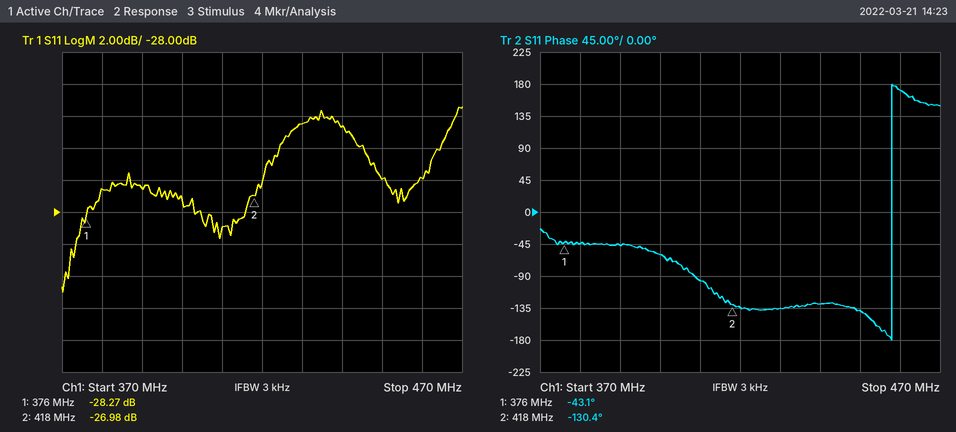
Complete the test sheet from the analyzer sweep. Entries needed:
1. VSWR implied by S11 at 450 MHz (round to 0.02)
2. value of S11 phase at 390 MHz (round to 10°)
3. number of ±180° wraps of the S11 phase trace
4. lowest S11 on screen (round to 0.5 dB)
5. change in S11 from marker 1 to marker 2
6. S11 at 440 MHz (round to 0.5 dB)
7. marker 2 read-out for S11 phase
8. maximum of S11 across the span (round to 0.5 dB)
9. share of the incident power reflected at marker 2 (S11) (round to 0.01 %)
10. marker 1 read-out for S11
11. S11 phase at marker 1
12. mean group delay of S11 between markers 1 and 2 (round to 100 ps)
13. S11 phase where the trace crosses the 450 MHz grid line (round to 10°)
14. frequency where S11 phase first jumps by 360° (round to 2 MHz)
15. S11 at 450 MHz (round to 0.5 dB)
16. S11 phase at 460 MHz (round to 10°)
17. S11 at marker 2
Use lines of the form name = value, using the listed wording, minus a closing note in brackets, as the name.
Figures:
VSWR implied by S11 at 450 MHz = 1.10
value of S11 phase at 390 MHz = -50°
number of ±180° wraps of the S11 phase trace = 1
lowest S11 on screen = -33.0 dB
change in S11 from marker 1 to marker 2 = 1.29 dB
S11 at 440 MHz = -22.5 dB
marker 2 read-out for S11 phase = -130.4°
maximum of S11 across the span = -21.5 dB
share of the incident power reflected at marker 2 (S11) = 0.20 %
marker 1 read-out for S11 = -28.27 dB
S11 phase at marker 1 = -43.1°
mean group delay of S11 between markers 1 and 2 = 5.8 ns
S11 phase where the trace crosses the 450 MHz grid line = -140°
frequency where S11 phase first jumps by 360° = 458 MHz
S11 at 450 MHz = -26.0 dB
S11 phase at 460 MHz = 170°
S11 at marker 2 = -26.98 dB
